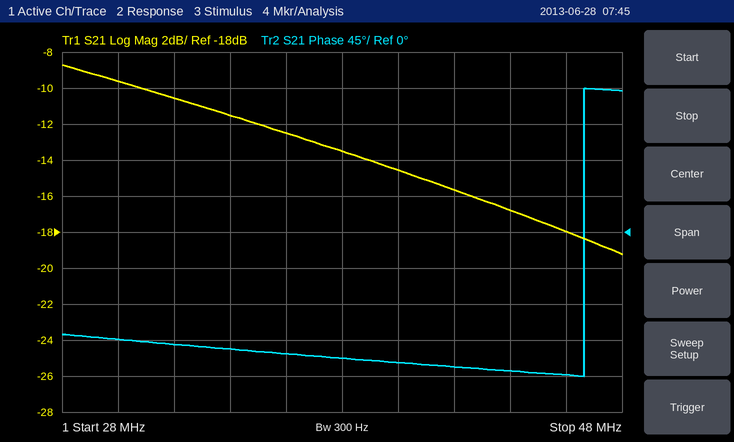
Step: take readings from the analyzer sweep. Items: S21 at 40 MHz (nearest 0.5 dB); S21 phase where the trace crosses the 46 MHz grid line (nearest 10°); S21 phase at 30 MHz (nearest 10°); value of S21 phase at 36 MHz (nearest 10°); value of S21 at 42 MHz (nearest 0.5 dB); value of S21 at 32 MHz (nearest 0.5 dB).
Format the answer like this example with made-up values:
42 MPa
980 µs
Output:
-14.5 dB
-180°
-130°
-150°
-15.5 dB
-10.5 dB
